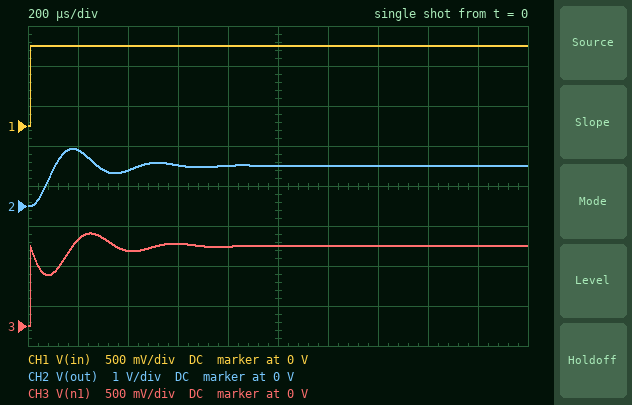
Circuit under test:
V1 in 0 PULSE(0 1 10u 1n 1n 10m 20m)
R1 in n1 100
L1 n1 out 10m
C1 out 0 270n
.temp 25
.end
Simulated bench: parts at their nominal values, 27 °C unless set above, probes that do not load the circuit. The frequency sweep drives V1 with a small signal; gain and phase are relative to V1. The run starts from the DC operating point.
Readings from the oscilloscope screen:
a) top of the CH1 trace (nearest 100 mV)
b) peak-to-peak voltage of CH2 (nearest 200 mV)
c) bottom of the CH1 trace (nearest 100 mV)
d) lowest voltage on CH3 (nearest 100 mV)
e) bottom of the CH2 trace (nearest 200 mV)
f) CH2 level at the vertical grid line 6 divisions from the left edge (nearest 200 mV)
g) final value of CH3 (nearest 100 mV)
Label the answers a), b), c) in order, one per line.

a) 1.0 V
b) 1.4 V
c) 0 V
d) 0 V
e) 0 V
f) 1.0 V
g) 1.0 V
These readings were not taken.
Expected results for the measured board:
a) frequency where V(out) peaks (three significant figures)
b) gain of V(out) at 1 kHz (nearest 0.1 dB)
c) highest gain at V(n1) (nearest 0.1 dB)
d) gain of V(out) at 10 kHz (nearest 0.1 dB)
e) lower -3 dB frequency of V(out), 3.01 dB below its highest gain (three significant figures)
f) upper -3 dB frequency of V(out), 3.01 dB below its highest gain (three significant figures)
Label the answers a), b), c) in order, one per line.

a) 2.85 kHz
b) 0.8 dB
c) 0 dB
d) -19.8 dB
e) 1.85 kHz
f) 3.58 kHz
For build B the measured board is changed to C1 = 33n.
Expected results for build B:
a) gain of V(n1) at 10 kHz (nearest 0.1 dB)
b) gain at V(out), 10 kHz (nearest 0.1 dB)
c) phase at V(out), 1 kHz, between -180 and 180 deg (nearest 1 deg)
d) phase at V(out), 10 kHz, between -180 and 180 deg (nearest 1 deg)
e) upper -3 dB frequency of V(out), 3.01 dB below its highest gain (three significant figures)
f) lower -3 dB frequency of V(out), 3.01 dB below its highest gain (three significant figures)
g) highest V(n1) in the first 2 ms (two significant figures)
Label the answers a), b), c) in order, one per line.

a) -1.7 dB
b) 8.7 dB
c) -1 deg
d) -146 deg
e) 9.45 kHz
f) 7.85 kHz
g) 1.1 V
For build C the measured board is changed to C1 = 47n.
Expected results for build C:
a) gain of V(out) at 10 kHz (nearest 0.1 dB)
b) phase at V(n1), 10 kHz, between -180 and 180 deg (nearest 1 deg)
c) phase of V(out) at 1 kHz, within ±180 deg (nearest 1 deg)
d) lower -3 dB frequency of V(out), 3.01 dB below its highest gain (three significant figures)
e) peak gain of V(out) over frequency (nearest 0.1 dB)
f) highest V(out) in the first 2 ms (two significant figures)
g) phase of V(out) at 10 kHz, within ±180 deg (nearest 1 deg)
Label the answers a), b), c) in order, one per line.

a) 0.9 dB
b) 19 deg
c) -2 deg
d) 6.40 kHz
e) 13.3 dB
f) 1.7 V
g) -161 deg
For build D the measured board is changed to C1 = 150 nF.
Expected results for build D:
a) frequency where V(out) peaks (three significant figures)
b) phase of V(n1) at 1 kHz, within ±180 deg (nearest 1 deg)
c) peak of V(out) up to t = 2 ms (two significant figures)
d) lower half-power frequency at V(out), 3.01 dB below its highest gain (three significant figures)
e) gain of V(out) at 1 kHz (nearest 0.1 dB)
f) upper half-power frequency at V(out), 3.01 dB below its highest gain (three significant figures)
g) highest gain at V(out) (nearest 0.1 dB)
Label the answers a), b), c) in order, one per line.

a) 3.95 kHz
b) -6 deg
c) 1.5 V
d) 3.03 kHz
e) 0.5 dB
f) 4.69 kHz
g) 8.4 dB
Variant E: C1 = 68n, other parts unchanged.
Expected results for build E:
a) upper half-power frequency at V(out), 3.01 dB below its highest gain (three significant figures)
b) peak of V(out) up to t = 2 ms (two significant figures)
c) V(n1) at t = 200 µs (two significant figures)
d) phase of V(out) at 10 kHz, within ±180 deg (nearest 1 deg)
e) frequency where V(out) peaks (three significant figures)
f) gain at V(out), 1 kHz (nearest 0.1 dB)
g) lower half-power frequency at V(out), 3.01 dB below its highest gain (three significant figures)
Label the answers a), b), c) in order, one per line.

a) 6.75 kHz
b) 1.7 V
c) 920 mV
d) -166 deg
e) 6.00 kHz
f) 0.2 dB
g) 5.13 kHz
